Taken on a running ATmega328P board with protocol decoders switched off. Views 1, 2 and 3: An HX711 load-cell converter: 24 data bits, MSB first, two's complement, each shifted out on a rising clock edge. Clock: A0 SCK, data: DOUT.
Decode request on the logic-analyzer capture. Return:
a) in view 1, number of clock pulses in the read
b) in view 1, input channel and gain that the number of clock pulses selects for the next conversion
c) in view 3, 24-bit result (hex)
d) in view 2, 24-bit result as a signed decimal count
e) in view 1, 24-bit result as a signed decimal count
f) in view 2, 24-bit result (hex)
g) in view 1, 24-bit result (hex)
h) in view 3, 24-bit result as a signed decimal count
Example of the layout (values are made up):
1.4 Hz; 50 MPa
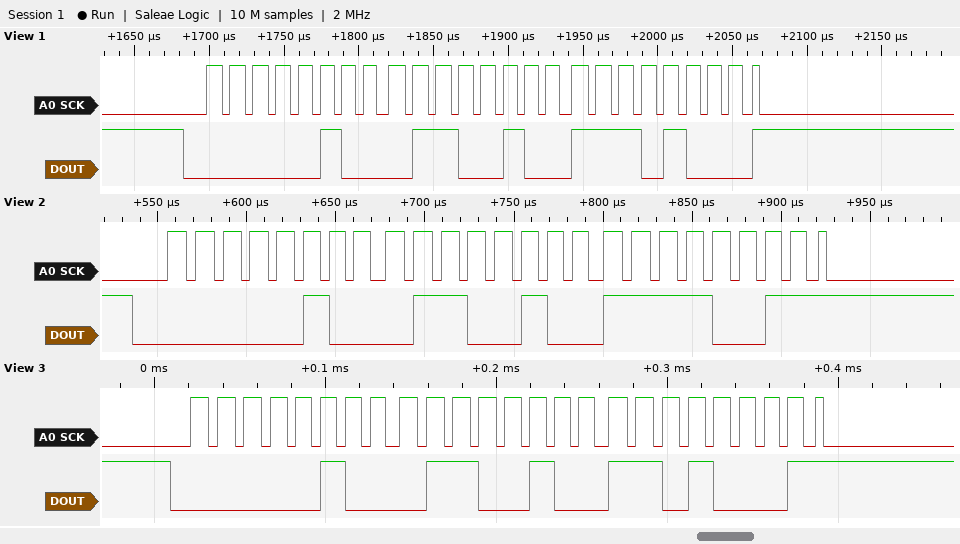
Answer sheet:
25; channel A, gain 128; 0x0464D1; 287987; 287976; 0x0464F3; 0x0464E8; 287953
